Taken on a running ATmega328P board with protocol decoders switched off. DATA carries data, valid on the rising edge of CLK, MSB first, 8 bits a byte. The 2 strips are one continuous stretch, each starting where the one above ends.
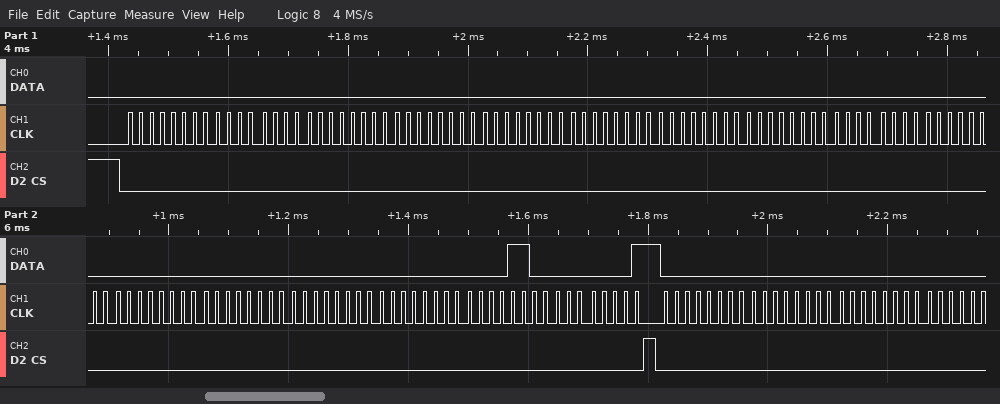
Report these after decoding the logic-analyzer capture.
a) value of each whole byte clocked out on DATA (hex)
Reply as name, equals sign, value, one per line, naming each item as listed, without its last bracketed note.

value of each whole byte clocked out on DATA = 00 00 00 00 00 00 00 00 00 00 00 00 00 00 0C 01 00 00 00
